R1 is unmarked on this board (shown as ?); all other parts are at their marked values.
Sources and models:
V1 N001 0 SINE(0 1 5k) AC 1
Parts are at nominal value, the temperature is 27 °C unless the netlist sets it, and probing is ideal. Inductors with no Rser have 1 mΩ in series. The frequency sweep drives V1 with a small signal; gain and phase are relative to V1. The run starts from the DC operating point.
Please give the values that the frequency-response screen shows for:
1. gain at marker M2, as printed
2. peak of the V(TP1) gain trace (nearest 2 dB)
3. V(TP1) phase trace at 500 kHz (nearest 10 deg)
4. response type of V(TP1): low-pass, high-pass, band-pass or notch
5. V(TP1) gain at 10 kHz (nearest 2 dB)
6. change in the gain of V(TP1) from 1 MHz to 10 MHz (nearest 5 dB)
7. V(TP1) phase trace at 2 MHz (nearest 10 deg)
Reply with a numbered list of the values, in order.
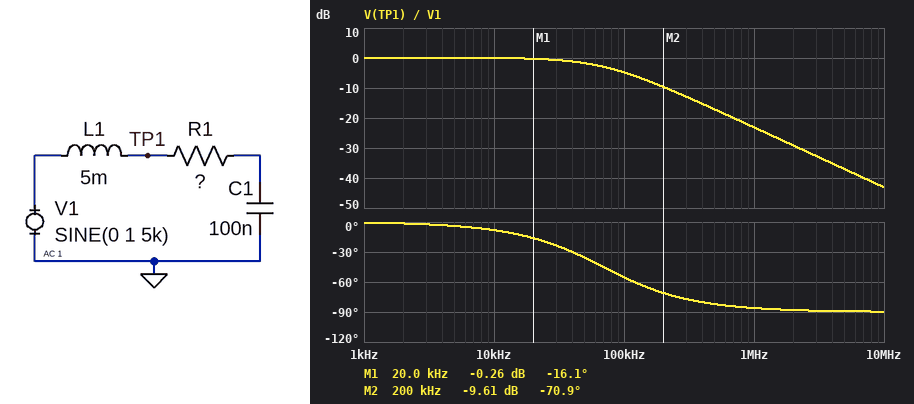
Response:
1. -9.61 dB
2. 0 dB
3. -80 deg
4. low-pass
5. 0 dB
6. -20 dB
7. -90 deg
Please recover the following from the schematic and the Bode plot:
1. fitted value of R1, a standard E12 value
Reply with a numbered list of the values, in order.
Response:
1. 2.2 kΩ
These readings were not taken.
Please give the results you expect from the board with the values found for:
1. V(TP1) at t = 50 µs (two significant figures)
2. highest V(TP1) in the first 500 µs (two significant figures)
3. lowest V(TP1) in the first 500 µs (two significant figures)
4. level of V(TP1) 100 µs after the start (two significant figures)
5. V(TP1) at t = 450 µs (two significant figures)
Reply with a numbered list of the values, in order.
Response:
1. 1.0 V
2. 1.0 V
3. -1.0 V
4. 70 mV
5. 1.0 V
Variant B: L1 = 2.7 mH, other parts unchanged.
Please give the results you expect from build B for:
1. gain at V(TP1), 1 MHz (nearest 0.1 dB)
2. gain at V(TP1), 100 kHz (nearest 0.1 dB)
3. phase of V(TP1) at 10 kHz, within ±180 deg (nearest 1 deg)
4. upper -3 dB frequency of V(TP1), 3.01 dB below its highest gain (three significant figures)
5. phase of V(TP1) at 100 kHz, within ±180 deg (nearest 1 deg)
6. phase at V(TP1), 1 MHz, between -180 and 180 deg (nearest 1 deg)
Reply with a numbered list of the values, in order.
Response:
1. -17.8 dB
2. -2.0 dB
3. -4 deg
4. 129 kHz
5. -38 deg
6. -83 deg
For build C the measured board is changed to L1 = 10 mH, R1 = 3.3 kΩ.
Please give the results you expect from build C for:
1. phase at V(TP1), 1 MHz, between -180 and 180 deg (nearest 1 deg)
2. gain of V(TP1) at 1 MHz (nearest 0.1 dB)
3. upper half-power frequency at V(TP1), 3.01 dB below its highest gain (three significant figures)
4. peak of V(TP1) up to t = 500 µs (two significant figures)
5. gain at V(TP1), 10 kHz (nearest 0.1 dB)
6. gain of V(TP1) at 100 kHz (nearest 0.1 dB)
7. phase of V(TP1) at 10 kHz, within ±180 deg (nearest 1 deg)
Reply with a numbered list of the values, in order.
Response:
1. -87 deg
2. -25.6 dB
3. 52.2 kHz
4. 1.0 V
5. -0.1 dB
6. -6.6 dB
7. -11 deg
